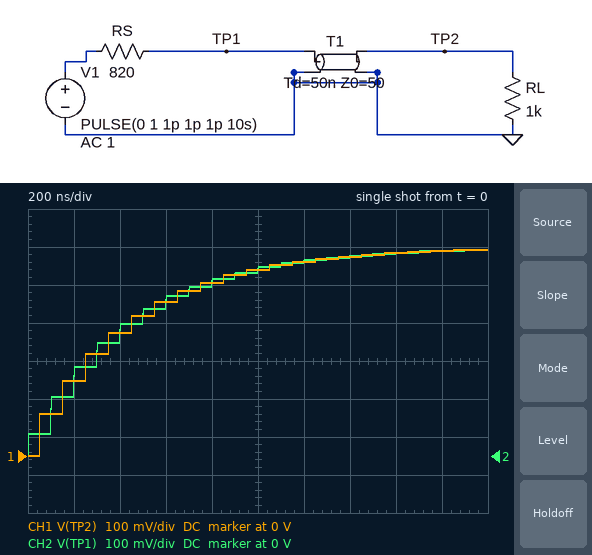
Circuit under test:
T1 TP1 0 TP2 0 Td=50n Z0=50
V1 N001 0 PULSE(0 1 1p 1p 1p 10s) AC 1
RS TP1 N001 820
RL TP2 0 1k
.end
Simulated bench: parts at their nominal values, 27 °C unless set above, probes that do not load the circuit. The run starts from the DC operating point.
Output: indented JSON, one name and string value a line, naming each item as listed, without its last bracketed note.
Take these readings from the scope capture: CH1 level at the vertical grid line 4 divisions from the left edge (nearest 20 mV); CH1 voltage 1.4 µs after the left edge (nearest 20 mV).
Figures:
{
  "CH1 level at the vertical grid line 4 divisions from the left edge": "460 mV",
  "CH1 voltage 1.4 µs after the left edge": "520 mV"
}
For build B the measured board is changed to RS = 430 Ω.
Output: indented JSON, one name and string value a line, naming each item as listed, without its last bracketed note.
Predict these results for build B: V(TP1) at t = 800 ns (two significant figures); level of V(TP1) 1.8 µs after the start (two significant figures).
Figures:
{
  "V(TP1) at t = 800 ns": "650 mV",
  "level of V(TP1) 1.8 µs after the start": "700 mV"
}
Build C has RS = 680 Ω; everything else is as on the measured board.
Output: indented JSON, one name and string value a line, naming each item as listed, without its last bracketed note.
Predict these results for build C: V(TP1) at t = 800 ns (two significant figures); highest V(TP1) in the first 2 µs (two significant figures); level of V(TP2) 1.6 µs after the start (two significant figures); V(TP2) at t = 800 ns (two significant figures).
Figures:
{
  "V(TP1) at t = 800 ns": "520 mV",
  "highest V(TP1) in the first 2 µs": "590 mV",
  "level of V(TP2) 1.6 µs after the start": "580 mV",
  "V(TP2) at t = 800 ns": "510 mV"
}
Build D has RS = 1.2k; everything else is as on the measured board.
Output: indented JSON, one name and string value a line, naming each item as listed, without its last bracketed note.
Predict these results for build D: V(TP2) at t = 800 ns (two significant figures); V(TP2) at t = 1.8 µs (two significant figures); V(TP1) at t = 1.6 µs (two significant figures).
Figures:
{
  "V(TP2) at t = 800 ns": "350 mV",
  "V(TP2) at t = 1.8 µs": "440 mV",
  "V(TP1) at t = 1.6 µs": "430 mV"
}
